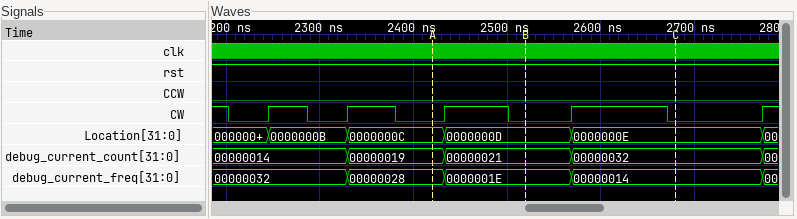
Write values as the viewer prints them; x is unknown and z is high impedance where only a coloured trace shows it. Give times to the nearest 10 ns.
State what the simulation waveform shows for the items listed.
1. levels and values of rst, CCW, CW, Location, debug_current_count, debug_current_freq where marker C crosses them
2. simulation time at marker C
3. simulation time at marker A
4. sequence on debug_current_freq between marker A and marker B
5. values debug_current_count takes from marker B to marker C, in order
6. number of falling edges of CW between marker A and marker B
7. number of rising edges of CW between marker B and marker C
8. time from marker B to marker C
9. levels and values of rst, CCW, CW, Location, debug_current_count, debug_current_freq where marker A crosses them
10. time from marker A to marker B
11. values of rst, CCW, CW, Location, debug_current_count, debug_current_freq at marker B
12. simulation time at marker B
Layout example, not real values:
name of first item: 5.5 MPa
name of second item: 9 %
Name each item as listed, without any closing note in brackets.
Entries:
levels and values of rst, CCW, CW, Location, debug_current_count, debug_current_freq where marker C crosses them: rst=1, CCW=0, CW=0, Location=0000000E, debug_current_count=00000032, debug_current_freq=00000014
simulation time at marker C: 2680 ns
simulation time at marker A: 2420 ns
sequence on debug_current_freq between marker A and marker B: 00000028, 0000001E
values debug_current_count takes from marker B to marker C, in order: 00000021, 00000032
number of falling edges of CW between marker A and marker B: 1
number of rising edges of CW between marker B and marker C: 1
time from marker B to marker C: 160 ns
levels and values of rst, CCW, CW, Location, debug_current_count, debug_current_freq where marker A crosses them: rst=1, CCW=0, CW=0, Location=0000000C, debug_current_count=00000019, debug_current_freq=00000028
time from marker A to marker B: 100 ns
values of rst, CCW, CW, Location, debug_current_count, debug_current_freq at marker B: rst=1, CCW=0, CW=0, Location=0000000D, debug_current_count=00000021, debug_current_freq=0000001E
simulation time at marker B: 2520 ns
